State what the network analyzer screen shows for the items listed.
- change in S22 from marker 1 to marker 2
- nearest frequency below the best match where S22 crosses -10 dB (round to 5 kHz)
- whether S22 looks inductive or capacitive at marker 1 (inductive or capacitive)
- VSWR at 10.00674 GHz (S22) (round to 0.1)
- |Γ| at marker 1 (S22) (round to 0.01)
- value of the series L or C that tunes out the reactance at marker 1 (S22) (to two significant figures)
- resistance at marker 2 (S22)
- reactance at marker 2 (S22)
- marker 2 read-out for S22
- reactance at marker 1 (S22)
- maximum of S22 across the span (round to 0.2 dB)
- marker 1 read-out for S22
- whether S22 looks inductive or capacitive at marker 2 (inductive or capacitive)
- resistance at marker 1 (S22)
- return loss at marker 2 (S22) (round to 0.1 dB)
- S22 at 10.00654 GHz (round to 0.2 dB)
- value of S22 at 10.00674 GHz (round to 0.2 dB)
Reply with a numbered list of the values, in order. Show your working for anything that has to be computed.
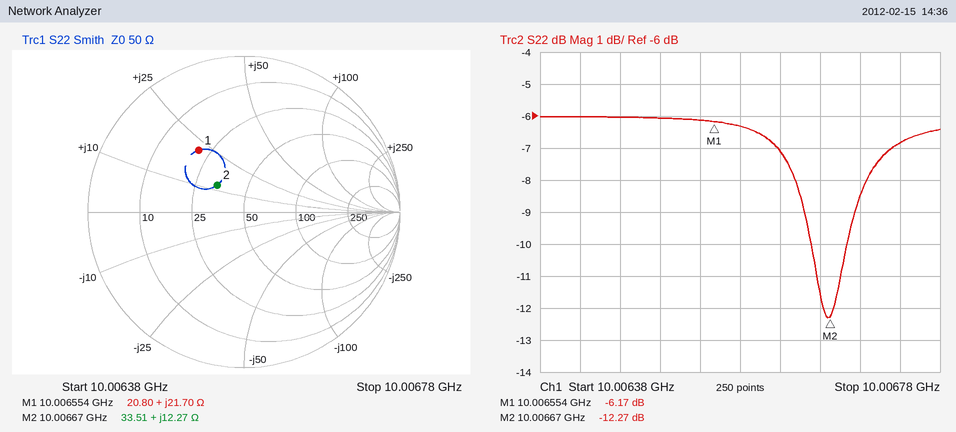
1. -12.27 − (-6.17) = -6.10 dB
2. 10.006650 GHz
3. inductive
4. |Γ| = 10^(-6.8/20) = 0.4571; VSWR = (1 + 0.4571)/(1 − 0.4571) ≈ 2.7
5. 0.49
6. C = 1/(2π × 10.006554 GHz × 21.7 Ω) ≈ 733 fF, so 730 fF to two significant figures
7. 33.51 Ω
8. +12.27 Ω
9. -12.27 dB
10. +21.70 Ω
11. -6.0 dB
12. -6.17 dB
13. inductive
14. 20.80 Ω
15. 12.3 dB
16. -6.2 dB
17. -6.8 dB
